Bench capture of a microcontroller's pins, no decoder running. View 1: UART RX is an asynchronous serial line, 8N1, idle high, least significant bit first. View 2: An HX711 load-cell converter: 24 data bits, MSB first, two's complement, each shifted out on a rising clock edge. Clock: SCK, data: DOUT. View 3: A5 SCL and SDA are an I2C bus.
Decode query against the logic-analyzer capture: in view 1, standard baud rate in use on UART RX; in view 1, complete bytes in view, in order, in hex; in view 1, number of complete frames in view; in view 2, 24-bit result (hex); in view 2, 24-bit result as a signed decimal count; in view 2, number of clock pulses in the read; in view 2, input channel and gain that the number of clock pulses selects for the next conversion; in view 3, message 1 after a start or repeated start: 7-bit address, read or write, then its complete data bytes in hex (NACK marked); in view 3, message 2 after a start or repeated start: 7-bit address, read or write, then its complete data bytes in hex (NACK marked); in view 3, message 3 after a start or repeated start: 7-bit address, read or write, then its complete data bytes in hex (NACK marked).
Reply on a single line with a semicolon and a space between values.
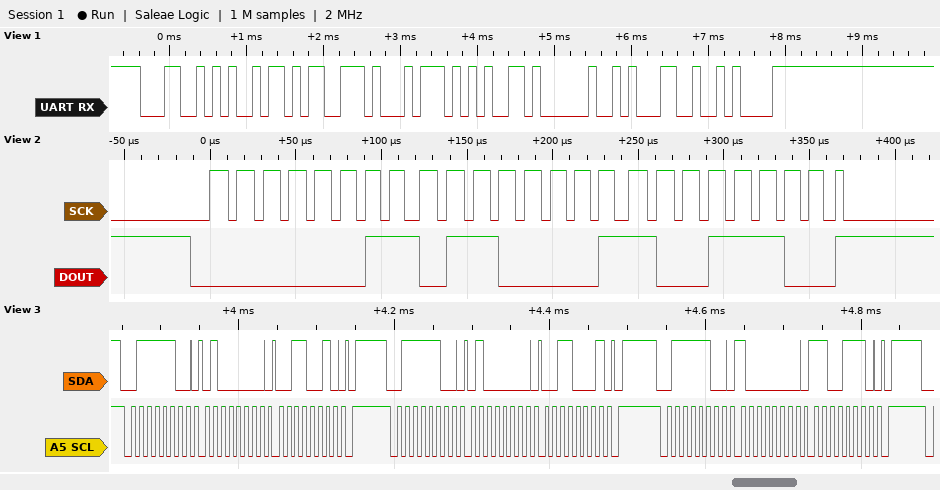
9600 baud; 0x4C 0x69 0x73 0x74 0x65 0x20 0x31 0x0A; 8; 0x03619C; 221596; 25; channel A, gain 128; 0x3E write: 40 32; 0x3E write: 40 31; 0x3E write: 80 CE
